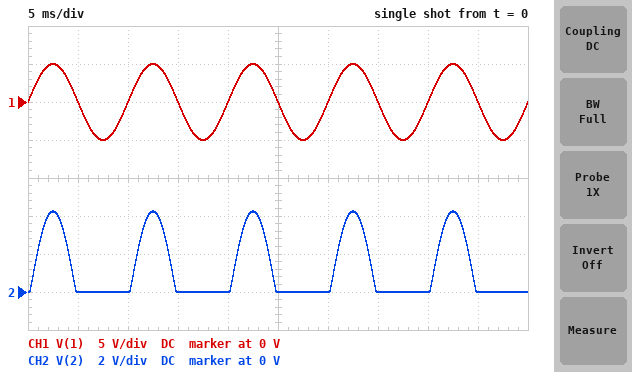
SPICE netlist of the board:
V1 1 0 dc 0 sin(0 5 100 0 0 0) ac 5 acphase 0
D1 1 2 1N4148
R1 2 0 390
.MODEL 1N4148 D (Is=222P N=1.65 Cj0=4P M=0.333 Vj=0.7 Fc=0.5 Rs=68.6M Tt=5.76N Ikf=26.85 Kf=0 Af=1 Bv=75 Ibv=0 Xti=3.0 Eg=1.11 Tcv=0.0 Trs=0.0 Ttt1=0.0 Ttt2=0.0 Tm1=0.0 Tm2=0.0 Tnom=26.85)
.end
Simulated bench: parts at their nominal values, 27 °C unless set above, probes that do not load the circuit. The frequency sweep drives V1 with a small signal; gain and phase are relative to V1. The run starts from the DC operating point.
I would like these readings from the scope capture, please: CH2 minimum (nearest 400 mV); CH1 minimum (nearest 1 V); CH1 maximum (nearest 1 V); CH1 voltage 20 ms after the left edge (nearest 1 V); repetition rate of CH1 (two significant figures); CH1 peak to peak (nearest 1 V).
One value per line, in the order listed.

0 V
-5 V
5 V
0 V
100 Hz
10 V
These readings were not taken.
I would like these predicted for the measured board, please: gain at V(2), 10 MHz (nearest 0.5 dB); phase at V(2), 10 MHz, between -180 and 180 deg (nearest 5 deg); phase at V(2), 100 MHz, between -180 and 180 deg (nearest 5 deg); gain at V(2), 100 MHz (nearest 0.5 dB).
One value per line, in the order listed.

-20.0 dB
85 deg
45 deg
-3.0 dB
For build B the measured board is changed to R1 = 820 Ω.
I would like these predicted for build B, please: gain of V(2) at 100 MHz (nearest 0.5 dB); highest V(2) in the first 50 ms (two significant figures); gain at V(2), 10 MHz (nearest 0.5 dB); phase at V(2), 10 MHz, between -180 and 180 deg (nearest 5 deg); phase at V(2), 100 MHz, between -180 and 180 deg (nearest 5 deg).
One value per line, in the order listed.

-1.0 dB
4.3 V
-14.0 dB
80 deg
25 deg
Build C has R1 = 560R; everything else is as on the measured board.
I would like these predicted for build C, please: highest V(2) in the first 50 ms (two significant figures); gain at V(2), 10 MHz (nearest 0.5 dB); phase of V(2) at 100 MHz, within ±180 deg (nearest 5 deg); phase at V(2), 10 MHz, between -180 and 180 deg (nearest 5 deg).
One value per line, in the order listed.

4.3 V
-17.0 dB
35 deg
80 deg
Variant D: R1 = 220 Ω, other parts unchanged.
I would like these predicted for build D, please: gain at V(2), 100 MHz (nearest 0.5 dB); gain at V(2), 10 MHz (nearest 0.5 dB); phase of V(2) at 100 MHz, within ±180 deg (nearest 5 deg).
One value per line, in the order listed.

-6.5 dB
-25.0 dB
60 deg
